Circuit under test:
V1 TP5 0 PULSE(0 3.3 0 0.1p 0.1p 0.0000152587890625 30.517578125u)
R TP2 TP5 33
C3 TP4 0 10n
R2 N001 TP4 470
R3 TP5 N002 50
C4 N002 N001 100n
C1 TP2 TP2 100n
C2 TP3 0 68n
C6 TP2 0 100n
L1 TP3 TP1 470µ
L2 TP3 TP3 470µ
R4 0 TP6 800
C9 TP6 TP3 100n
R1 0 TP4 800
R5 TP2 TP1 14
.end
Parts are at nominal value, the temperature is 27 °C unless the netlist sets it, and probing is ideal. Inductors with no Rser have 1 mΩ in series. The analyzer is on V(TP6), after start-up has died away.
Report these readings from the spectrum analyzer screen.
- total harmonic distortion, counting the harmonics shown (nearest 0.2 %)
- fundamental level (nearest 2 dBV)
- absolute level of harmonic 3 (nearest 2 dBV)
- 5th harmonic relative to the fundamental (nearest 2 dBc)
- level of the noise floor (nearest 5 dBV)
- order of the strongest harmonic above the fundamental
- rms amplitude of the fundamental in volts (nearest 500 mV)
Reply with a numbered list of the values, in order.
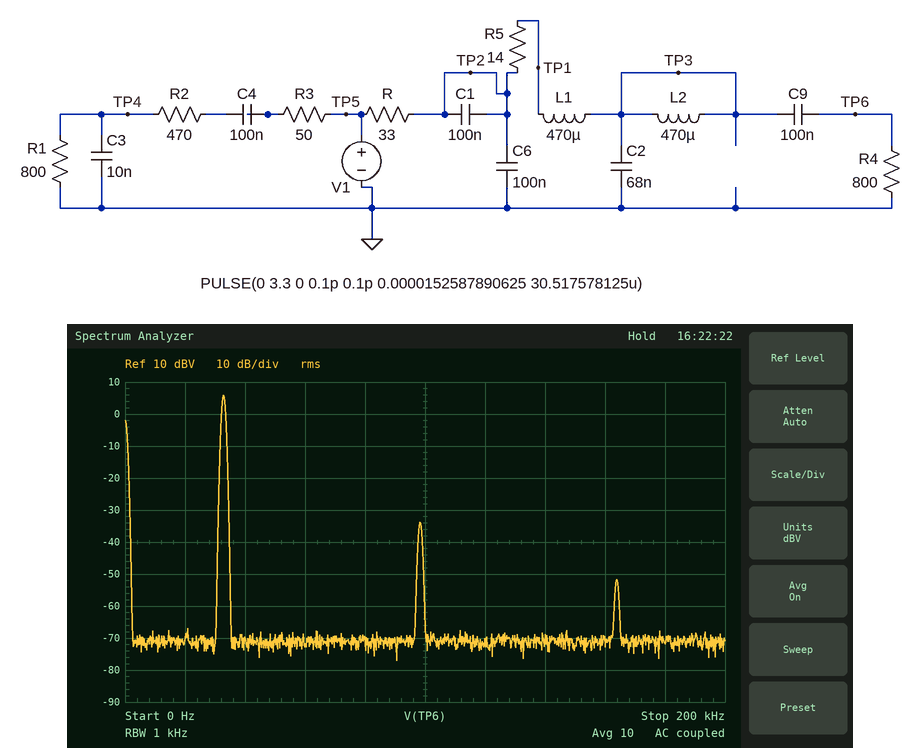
1. 1.0 %
2. 6 dBV
3. -34 dBV
4. -58 dBc
5. -70 dBV
6. 3
7. 2.0 V
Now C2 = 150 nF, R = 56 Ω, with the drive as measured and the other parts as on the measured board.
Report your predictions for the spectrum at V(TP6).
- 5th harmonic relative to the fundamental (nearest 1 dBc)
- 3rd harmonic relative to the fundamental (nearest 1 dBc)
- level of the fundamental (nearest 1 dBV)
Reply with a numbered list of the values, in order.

1. -58 dBc
2. -40 dBc
3. -5 dBV
